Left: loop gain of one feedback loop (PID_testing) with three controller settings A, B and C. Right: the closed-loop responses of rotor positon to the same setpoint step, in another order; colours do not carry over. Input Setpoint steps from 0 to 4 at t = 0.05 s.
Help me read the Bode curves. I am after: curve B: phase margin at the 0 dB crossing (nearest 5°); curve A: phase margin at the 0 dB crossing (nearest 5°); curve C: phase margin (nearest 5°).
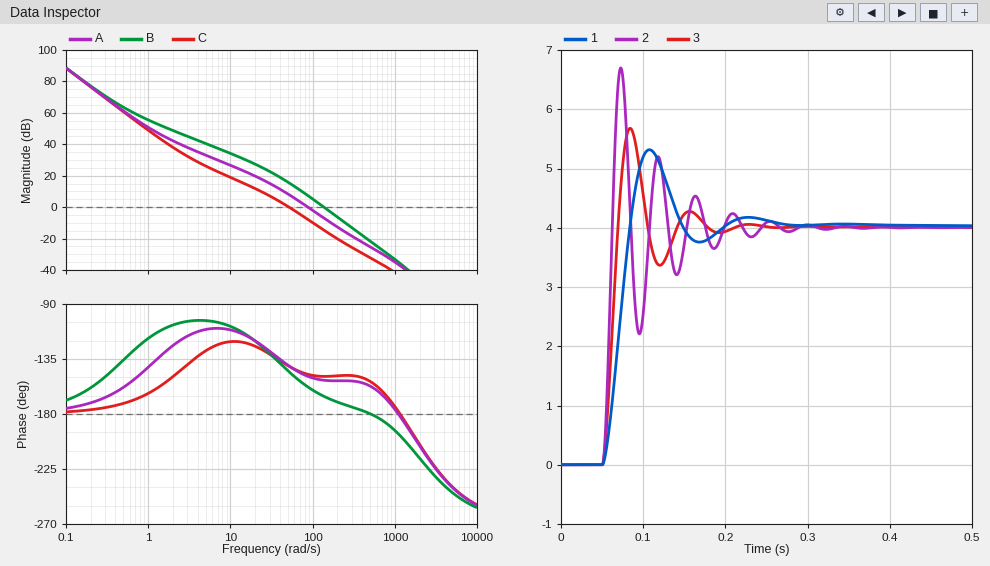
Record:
15°
30°
40°
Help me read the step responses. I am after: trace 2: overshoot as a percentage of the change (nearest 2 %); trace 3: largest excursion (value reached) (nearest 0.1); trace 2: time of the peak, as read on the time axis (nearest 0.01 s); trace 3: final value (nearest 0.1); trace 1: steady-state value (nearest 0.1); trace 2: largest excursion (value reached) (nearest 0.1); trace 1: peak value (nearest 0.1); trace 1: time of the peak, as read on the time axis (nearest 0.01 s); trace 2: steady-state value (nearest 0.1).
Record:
68 %
5.7
0.07 s
4.0
4.0
6.7
5.3
0.11 s
4.0
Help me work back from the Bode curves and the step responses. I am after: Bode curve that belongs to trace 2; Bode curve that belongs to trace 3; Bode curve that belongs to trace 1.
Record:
B
A
C
